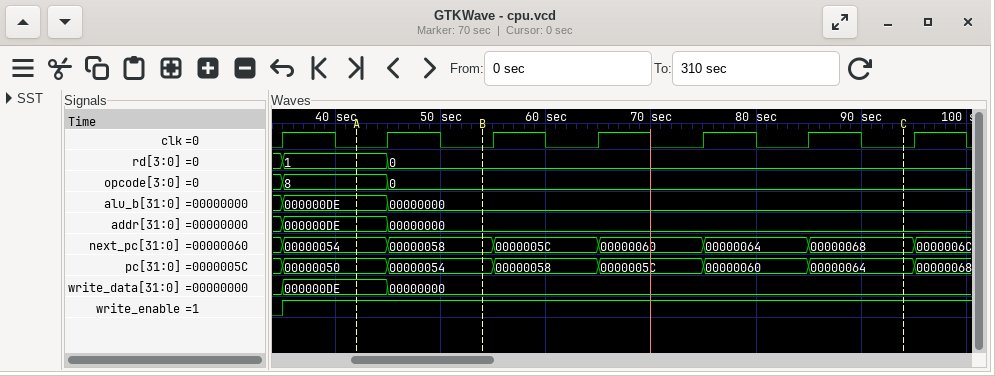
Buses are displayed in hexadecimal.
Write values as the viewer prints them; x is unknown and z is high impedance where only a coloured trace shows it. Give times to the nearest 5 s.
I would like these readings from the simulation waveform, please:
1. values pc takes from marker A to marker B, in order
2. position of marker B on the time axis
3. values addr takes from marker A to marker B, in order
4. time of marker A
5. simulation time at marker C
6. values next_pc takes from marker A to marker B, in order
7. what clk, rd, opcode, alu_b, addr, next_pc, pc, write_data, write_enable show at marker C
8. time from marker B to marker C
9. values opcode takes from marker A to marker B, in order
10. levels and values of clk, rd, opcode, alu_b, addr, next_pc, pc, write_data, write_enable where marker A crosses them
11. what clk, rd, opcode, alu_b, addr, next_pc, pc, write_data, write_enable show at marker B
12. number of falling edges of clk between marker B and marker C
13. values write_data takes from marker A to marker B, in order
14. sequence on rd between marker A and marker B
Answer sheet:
00000050, 00000054
55 s
000000DE, 00000000
40 s
95 s
00000054, 00000058
clk=0, rd=0, opcode=0, alu_b=00000000, addr=00000000, next_pc=00000068, pc=00000064, write_data=00000000, write_enable=1
40 s
8, 0
clk=0, rd=1, opcode=8, alu_b=000000DE, addr=000000DE, next_pc=00000054, pc=00000050, write_data=000000DE, write_enable=1
clk=0, rd=0, opcode=0, alu_b=00000000, addr=00000000, next_pc=00000058, pc=00000054, write_data=00000000, write_enable=1
4
000000DE, 00000000
1, 0
